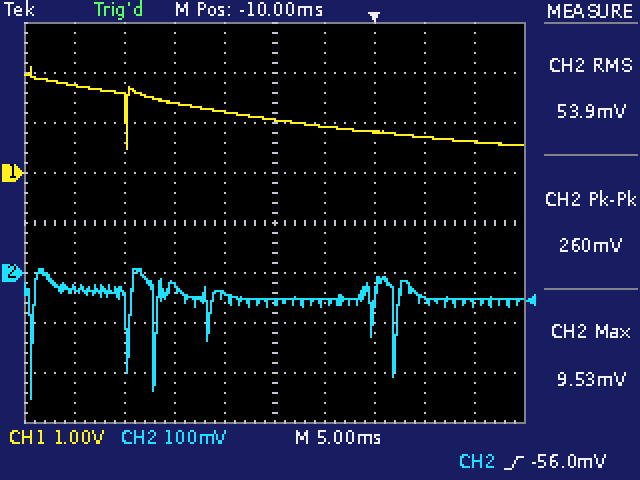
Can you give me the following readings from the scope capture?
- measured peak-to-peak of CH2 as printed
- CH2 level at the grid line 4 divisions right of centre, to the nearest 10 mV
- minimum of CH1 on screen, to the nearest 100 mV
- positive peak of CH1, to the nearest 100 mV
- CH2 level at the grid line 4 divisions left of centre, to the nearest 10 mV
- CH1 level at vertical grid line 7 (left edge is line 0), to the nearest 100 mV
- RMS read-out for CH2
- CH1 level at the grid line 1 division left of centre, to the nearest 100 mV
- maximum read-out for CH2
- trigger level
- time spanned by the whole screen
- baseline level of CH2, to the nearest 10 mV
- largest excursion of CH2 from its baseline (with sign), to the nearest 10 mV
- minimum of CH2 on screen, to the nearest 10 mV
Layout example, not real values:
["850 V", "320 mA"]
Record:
["260 mV", "-60 mV", "500 mV", "2.1 V", "-30 mV", "800 mV", "53.9 mV", "1.2 V", "9.53 mV", "-56.0 mV", "50 ms", "-50 mV", "-200 mV", "-250 mV"]
